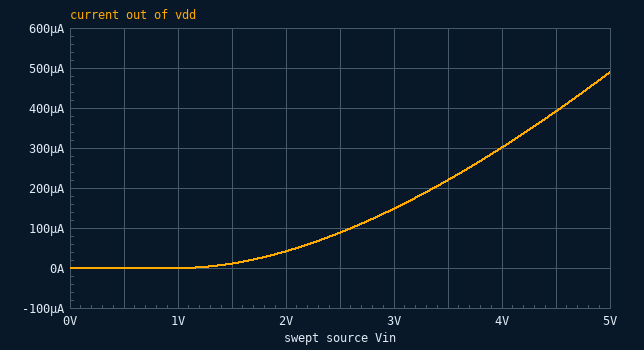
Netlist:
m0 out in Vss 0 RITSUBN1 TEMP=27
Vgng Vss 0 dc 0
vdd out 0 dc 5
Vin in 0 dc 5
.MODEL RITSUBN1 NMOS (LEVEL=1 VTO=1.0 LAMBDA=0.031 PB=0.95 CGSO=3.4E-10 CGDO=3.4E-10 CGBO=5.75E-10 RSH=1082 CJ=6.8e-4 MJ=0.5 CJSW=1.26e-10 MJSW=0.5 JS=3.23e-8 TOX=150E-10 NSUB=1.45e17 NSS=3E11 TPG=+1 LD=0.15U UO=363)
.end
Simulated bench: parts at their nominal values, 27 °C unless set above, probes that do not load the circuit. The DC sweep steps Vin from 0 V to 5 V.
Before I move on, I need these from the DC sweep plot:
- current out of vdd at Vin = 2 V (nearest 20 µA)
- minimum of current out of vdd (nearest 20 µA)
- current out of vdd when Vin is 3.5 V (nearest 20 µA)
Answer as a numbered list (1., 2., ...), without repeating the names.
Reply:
1. 40 µA
2. 0 A
3. 220 µA
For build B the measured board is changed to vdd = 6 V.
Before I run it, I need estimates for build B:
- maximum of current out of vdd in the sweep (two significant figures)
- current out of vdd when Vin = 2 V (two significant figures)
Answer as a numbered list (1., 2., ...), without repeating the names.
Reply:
1. 500 µA
2. 43 µA
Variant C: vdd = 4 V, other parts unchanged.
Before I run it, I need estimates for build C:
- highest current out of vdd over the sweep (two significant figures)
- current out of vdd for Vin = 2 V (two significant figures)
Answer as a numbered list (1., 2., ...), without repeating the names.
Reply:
1. 480 µA
2. 41 µA
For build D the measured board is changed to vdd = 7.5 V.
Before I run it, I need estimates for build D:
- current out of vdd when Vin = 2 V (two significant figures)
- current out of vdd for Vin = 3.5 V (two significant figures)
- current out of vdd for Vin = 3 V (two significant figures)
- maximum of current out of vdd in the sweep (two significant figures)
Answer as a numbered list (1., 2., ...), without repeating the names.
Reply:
1. 44 µA
2. 230 µA
3. 160 µA
4. 510 µA
